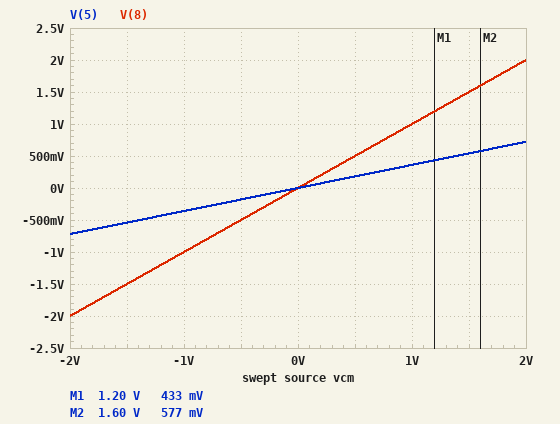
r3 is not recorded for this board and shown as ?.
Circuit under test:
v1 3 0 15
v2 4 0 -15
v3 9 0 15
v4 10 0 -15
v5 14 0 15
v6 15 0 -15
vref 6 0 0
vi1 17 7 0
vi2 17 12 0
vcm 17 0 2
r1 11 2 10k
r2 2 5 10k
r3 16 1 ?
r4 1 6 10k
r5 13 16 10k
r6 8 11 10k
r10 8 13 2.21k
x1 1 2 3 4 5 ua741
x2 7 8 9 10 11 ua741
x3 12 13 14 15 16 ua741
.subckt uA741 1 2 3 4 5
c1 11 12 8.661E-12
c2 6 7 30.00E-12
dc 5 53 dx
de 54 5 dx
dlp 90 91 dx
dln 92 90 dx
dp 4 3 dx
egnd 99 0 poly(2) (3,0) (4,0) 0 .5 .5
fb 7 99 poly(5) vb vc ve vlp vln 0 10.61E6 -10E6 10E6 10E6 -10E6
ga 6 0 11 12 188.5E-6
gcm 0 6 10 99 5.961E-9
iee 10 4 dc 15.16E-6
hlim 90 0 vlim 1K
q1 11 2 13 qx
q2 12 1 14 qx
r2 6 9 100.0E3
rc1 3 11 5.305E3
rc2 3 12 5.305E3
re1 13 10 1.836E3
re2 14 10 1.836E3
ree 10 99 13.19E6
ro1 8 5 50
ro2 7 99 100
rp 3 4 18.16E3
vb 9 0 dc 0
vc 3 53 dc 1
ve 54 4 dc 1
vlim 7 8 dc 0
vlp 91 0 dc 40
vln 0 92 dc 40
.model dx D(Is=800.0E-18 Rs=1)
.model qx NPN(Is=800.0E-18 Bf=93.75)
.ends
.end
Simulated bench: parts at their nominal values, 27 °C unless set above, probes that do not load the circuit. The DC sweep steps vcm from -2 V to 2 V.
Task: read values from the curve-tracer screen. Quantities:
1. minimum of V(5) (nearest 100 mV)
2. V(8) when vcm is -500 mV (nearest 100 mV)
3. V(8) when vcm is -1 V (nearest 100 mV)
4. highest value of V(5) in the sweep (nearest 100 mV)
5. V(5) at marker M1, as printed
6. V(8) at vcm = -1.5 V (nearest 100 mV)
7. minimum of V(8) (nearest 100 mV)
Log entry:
-700 mV
-500 mV
-1.0 V
700 mV
433 mV
-1.5 V
-2.0 V
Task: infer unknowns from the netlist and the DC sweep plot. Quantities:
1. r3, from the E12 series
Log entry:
4.7 kΩ
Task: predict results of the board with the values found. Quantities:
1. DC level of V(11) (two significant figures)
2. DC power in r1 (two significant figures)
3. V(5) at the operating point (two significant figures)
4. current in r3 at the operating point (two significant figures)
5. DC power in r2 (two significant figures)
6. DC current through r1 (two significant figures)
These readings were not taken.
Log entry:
2.0 V
41 µW
720 mV
140 µA
41 µW
64 µA
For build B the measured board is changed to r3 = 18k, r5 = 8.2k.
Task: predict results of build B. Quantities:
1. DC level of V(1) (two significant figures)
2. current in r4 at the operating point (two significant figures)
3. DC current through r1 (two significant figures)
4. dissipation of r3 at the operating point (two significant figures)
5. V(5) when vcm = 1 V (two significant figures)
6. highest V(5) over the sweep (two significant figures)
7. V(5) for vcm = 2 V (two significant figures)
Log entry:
710 mV
71 µA
130 µA
92 µW
-290 mV
570 mV
-570 mV
